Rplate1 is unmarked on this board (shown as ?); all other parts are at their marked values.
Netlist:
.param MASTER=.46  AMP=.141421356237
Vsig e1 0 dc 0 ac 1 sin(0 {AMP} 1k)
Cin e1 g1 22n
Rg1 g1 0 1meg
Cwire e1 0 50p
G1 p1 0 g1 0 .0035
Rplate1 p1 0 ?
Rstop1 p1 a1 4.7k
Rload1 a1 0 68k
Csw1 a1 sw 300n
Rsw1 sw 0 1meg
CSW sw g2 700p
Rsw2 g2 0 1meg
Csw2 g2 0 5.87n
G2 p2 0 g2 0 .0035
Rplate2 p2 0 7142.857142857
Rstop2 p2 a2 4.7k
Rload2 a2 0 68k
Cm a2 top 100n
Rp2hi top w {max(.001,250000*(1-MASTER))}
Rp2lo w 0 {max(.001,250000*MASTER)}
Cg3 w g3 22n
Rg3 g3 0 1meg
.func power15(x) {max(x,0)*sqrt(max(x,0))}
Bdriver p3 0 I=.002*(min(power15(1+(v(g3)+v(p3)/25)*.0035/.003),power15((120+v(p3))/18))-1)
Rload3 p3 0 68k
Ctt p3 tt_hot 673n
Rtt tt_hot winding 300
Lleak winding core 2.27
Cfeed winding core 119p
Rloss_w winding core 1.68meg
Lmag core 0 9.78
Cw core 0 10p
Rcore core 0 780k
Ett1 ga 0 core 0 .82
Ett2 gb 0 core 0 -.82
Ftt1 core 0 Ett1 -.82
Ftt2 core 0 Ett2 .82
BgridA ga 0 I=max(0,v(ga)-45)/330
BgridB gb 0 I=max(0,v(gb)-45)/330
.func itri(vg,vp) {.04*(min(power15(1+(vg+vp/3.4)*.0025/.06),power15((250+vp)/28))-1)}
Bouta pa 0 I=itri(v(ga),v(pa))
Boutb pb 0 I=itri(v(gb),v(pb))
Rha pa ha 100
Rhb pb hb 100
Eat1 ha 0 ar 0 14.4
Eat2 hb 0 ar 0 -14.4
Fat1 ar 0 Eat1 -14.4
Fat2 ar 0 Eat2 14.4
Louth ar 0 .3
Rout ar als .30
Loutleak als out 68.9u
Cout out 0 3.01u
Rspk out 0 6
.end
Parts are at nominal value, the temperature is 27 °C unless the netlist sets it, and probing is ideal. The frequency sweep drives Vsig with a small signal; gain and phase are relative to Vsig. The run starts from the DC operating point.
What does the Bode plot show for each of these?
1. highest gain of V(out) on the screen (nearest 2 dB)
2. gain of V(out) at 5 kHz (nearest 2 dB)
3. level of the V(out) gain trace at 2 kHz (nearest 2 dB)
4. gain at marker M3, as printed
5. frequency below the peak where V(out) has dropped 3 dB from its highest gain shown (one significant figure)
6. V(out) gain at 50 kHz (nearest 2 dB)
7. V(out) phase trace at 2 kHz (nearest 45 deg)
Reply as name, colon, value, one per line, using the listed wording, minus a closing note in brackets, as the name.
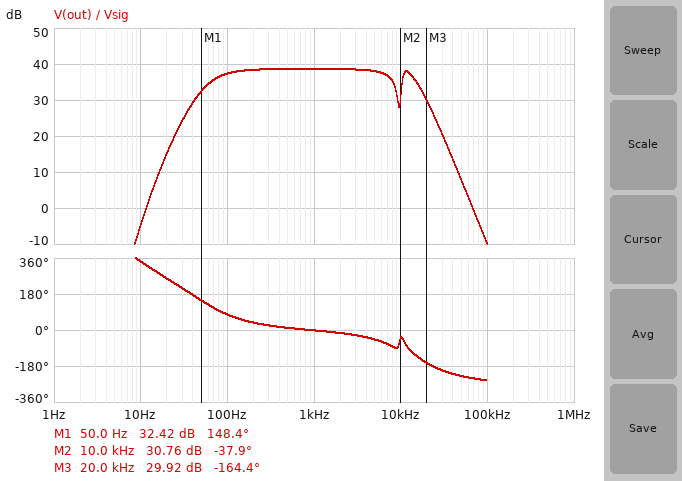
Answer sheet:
highest gain of V(out) on the screen: 38 dB
gain of V(out) at 5 kHz: 38 dB
level of the V(out) gain trace at 2 kHz: 38 dB
gain at marker M3, as printed: 29.92 dB
frequency below the peak where V(out) has dropped 3 dB from its highest gain shown: 70 Hz
V(out) gain at 50 kHz: 8 dB
V(out) phase trace at 2 kHz: 0 deg
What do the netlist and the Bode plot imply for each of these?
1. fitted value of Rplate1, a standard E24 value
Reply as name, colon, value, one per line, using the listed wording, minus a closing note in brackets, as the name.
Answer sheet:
fitted value of Rplate1, a standard E24 value: 16 kΩ
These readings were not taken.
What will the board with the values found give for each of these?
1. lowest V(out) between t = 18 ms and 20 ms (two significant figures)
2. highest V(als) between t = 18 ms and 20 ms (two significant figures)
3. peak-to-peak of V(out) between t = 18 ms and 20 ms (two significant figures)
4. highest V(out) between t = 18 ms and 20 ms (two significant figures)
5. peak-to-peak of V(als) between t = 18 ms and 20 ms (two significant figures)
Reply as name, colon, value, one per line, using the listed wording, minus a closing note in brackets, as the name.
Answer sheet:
lowest V(out) between t = 18 ms and 20 ms: -7.1 V
highest V(als) between t = 18 ms and 20 ms: 6.5 V
peak-to-peak of V(out) between t = 18 ms and 20 ms: 14 V
highest V(out) between t = 18 ms and 20 ms: 6.7 V
peak-to-peak of V(als) between t = 18 ms and 20 ms: 13 V
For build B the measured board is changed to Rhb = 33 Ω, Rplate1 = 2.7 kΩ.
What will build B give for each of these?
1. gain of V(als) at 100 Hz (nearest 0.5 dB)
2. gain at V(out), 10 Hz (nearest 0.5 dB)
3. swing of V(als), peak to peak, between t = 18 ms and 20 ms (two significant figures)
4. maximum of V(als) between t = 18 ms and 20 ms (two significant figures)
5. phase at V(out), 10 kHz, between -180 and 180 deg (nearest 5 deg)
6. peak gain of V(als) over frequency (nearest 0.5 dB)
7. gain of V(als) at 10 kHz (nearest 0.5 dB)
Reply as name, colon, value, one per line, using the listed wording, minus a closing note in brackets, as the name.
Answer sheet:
gain of V(als) at 100 Hz: 23.5 dB
gain at V(out), 10 Hz: -18.5 dB
swing of V(als), peak to peak, between t = 18 ms and 20 ms: 4.9 V
maximum of V(als) between t = 18 ms and 20 ms: 2.4 V
phase at V(out), 10 kHz, between -180 and 180 deg: -20 deg
peak gain of V(als) over frequency: 28.0 dB
gain of V(als) at 10 kHz: 15.5 dB
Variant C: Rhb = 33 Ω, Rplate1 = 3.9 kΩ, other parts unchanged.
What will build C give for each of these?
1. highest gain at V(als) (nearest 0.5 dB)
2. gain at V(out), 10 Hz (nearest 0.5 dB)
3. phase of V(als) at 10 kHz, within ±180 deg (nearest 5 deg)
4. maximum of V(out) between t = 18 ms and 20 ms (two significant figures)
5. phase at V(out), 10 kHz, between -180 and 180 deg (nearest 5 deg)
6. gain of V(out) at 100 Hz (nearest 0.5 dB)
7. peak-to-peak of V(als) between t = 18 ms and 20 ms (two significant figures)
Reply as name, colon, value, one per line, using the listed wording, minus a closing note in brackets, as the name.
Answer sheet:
highest gain at V(als): 30.5 dB
gain at V(out), 10 Hz: -15.5 dB
phase of V(als) at 10 kHz, within ±180 deg: 55 deg
maximum of V(out) between t = 18 ms and 20 ms: 3.5 V
phase at V(out), 10 kHz, between -180 and 180 deg: -25 deg
gain of V(out) at 100 Hz: 26.5 dB
peak-to-peak of V(als) between t = 18 ms and 20 ms: 6.9 V
